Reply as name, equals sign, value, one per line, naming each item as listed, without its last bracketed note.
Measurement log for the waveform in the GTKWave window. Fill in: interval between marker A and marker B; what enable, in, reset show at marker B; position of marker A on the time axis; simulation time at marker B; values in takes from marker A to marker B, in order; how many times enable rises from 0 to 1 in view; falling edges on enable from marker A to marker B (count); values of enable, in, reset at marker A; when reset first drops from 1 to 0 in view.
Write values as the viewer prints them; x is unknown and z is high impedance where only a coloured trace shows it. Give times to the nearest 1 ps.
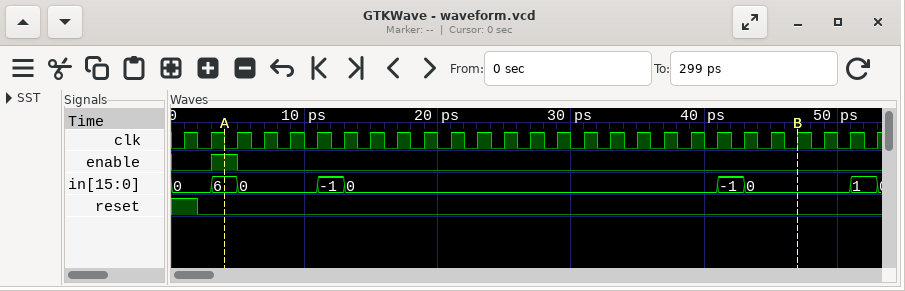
interval between marker A and marker B = 43 ps
what enable, in, reset show at marker B = enable=0, in=0, reset=0
position of marker A on the time axis = 4 ps
simulation time at marker B = 47 ps
values in takes from marker A to marker B, in order = 6, 0, -1, 0, -1, 0
how many times enable rises from 0 to 1 in view = 1
falling edges on enable from marker A to marker B = 1
values of enable, in, reset at marker A = enable=1, in=6, reset=0
when reset first drops from 1 to 0 in view = 2 ps
